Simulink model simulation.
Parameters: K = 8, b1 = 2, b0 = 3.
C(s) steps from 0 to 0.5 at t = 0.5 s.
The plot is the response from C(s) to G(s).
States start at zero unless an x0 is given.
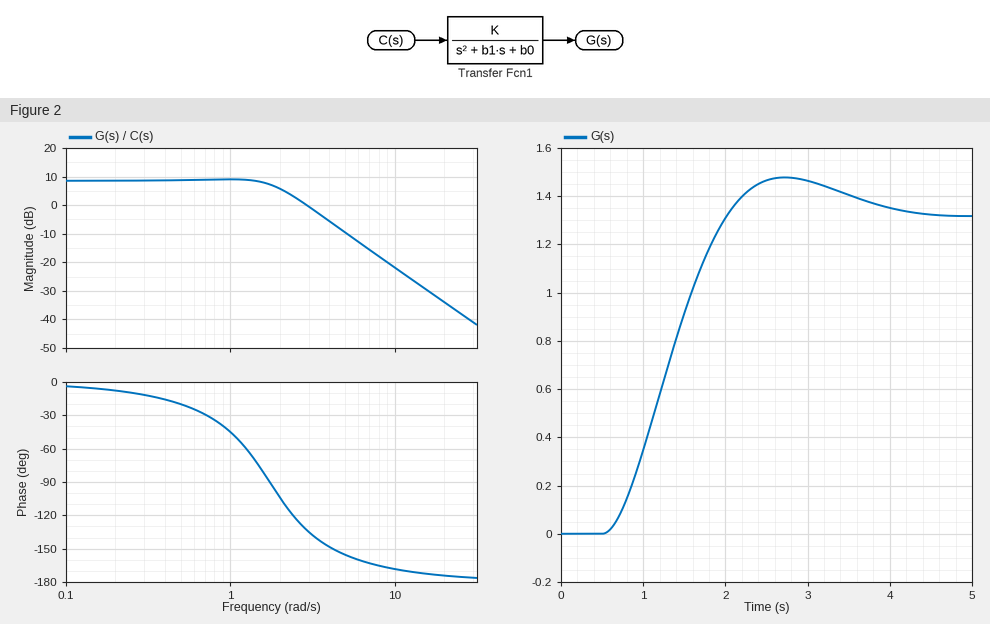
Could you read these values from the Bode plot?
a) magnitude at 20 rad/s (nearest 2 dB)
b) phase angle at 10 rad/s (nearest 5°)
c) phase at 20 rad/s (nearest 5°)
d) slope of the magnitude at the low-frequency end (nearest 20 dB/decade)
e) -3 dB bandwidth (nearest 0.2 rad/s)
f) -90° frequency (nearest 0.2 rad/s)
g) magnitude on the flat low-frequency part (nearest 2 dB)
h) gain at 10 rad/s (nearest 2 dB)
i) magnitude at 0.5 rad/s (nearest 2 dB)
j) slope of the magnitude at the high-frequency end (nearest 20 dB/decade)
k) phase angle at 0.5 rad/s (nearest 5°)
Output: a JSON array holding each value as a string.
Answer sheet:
["-34 dB", "-170°", "-175°", "0 dB/decade", "2.0 rad/s", "1.8 rad/s", "8 dB", "-22 dB", "8 dB", "-40 dB/decade", "-20°"]
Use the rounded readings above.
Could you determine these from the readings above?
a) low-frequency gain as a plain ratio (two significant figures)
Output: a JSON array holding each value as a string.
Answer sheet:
["2.5"]
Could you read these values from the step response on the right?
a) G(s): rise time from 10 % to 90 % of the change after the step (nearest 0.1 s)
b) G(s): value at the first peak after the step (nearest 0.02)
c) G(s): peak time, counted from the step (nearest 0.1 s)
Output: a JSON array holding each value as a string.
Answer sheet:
["1.0 s", "1.48", "2.2 s"]
